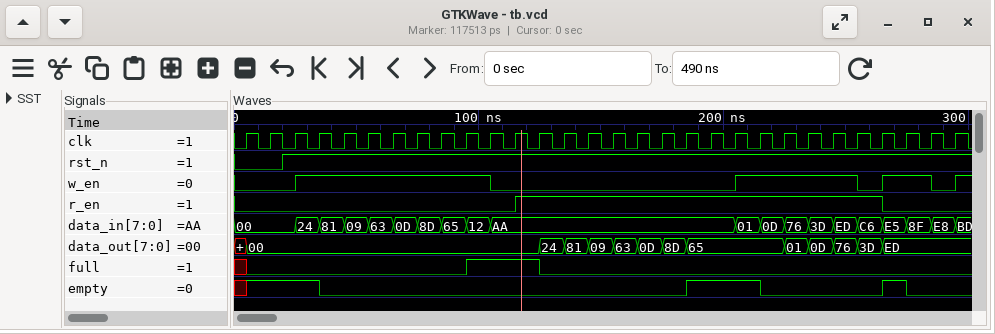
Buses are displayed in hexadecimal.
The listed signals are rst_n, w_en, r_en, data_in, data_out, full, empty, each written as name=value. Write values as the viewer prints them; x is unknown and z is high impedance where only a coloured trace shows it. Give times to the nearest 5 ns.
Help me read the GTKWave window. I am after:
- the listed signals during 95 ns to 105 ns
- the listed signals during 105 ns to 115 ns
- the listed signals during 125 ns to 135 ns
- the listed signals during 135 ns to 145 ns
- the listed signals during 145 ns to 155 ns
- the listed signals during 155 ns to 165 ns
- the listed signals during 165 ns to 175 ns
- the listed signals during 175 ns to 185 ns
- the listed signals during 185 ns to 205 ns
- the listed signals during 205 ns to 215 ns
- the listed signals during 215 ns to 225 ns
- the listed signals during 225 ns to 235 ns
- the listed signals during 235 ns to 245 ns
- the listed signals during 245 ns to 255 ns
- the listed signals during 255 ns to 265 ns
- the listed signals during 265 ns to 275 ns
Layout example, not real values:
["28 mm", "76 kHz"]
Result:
["rst_n=1, w_en=1, r_en=0, data_in=12, data_out=00, full=1, empty=0", "rst_n=1, w_en=0, r_en=0, data_in=AA, data_out=00, full=1, empty=0", "rst_n=1, w_en=0, r_en=1, data_in=AA, data_out=24, full=0, empty=0", "rst_n=1, w_en=0, r_en=1, data_in=AA, data_out=81, full=0, empty=0", "rst_n=1, w_en=0, r_en=1, data_in=AA, data_out=09, full=0, empty=0", "rst_n=1, w_en=0, r_en=1, data_in=AA, data_out=63, full=0, empty=0", "rst_n=1, w_en=0, r_en=1, data_in=AA, data_out=0D, full=0, empty=0", "rst_n=1, w_en=0, r_en=1, data_in=AA, data_out=8D, full=0, empty=0", "rst_n=1, w_en=0, r_en=1, data_in=AA, data_out=65, full=0, empty=1", "rst_n=1, w_en=1, r_en=1, data_in=01, data_out=65, full=0, empty=1", "rst_n=1, w_en=1, r_en=1, data_in=0D, data_out=65, full=0, empty=0", "rst_n=1, w_en=1, r_en=1, data_in=76, data_out=01, full=0, empty=0", "rst_n=1, w_en=1, r_en=1, data_in=3D, data_out=0D, full=0, empty=0", "rst_n=1, w_en=1, r_en=1, data_in=ED, data_out=76, full=0, empty=0", "rst_n=1, w_en=0, r_en=1, data_in=C6, data_out=3D, full=0, empty=0", "rst_n=1, w_en=1, r_en=0, data_in=E5, data_out=ED, full=0, empty=1"]
